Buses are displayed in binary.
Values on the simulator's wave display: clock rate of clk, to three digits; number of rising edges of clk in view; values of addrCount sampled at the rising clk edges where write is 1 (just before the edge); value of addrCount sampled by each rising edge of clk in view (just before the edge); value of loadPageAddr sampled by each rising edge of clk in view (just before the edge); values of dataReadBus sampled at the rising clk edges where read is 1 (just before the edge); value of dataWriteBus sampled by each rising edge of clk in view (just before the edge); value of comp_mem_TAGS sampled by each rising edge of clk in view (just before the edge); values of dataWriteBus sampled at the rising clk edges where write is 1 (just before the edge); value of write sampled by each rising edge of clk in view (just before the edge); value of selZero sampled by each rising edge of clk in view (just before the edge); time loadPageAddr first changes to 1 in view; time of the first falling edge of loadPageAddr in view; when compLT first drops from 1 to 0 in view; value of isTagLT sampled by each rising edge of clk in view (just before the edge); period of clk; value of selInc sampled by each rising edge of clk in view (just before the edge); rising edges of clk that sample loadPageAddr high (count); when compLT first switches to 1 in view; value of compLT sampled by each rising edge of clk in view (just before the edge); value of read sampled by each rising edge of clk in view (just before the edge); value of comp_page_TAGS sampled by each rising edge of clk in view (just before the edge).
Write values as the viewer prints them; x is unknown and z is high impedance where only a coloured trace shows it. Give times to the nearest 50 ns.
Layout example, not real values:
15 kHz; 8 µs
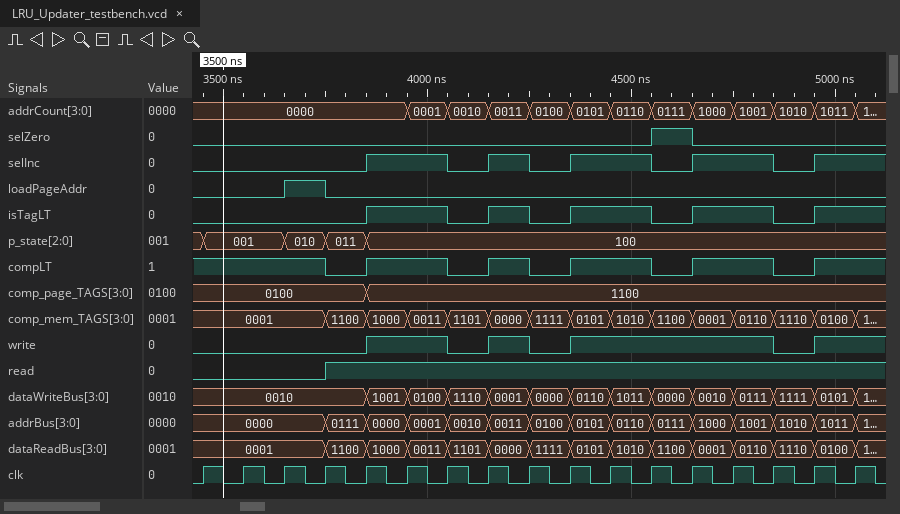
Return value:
10.0 MHz; 17; 0000, 0001, 0011, 0101, 0110, 0111, 1000, 1001, 1011; 0000, 0000, 0000, 0000, 0000, 0000, 0001, 0010, 0011, 0100, 0101, 0110, 0111, 1000, 1001, 1010, 1011; 0 0 0 1 0 0 0 0 0 0 0 0 0 0 0 0 0; 1100, 1000, 0011, 1101, 0000, 1111, 0101, 1010, 1100, 0001, 0110, 1110, 0100; 0010, 0010, 0010, 0010, 0010, 1001, 0100, 1110, 0001, 0000, 0110, 1011, 0000, 0010, 0111, 1111, 0101; 0001, 0001, 0001, 0001, 1100, 1000, 0011, 1101, 0000, 1111, 0101, 1010, 1100, 0001, 0110, 1110, 0100; 1001, 0100, 0001, 0110, 1011, 0000, 0010, 0111, 0101; 0 0 0 0 0 1 1 0 1 0 1 1 1 1 1 0 1; 0 0 0 0 0 0 0 0 0 0 0 0 1 0 0 0 0; 3650 ns; 3750 ns; 3750 ns; 0 0 0 0 0 1 1 0 1 0 1 1 0 1 1 0 1; 100 ns; 0 0 0 0 0 1 1 0 1 0 1 1 0 1 1 0 1; 1; 3850 ns; 1 1 1 1 0 1 1 0 1 0 1 1 0 1 1 0 1; 0 0 0 0 1 1 1 1 1 1 1 1 1 1 1 1 1; 0100, 0100, 0100, 0100, 0100, 1100, 1100, 1100, 1100, 1100, 1100, 1100, 1100, 1100, 1100, 1100, 1100
